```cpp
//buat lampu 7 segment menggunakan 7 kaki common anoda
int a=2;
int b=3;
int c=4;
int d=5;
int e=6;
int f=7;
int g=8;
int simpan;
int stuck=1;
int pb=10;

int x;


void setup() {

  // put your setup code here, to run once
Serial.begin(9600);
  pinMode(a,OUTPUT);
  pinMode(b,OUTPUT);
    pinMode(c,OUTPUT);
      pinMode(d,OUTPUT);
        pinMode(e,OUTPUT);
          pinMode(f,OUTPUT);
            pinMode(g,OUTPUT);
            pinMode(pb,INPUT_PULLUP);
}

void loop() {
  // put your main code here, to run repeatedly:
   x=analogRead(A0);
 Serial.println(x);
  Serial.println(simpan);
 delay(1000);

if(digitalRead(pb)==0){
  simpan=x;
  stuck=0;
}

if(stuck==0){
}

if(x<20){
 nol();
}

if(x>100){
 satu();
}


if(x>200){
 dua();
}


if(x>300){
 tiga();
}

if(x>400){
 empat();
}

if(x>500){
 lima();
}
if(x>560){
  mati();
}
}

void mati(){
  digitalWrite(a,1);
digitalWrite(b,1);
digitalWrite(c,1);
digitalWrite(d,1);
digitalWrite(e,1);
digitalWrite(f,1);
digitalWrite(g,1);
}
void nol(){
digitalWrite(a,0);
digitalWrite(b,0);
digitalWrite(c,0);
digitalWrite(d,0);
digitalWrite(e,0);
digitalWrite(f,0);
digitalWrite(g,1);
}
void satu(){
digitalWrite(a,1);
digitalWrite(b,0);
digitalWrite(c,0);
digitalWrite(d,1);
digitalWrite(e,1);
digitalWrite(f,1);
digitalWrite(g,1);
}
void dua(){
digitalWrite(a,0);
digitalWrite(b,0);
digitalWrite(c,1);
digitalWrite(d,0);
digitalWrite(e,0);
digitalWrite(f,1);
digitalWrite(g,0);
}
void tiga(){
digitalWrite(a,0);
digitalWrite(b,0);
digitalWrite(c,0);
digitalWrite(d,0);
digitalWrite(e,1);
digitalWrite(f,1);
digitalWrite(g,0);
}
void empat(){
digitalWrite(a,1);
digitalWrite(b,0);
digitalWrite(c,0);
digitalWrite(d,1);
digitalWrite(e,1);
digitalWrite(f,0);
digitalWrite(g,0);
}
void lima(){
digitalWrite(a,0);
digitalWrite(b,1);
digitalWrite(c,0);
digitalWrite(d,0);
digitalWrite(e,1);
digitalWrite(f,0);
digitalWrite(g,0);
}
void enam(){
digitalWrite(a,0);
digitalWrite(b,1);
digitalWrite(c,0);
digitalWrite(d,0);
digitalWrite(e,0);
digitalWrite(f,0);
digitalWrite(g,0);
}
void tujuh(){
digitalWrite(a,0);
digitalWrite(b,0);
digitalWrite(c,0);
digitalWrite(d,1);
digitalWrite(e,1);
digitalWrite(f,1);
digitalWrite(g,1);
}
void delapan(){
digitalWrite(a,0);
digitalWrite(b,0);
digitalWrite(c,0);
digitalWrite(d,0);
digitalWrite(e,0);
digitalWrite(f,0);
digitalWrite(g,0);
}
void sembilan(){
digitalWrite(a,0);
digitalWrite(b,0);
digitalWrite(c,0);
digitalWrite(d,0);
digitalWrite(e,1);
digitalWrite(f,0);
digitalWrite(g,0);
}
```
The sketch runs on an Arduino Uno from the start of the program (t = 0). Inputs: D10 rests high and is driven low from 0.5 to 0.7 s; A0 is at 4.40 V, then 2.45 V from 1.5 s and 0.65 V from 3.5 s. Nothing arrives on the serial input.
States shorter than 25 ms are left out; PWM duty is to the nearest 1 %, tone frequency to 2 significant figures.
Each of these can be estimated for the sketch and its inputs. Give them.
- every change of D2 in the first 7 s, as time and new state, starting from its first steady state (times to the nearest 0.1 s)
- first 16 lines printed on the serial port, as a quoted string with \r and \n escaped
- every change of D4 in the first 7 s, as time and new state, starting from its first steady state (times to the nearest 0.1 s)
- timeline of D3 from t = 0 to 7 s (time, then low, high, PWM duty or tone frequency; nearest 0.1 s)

0 s low; 1 s high; 3 s low; 5 s high
"901\r\n0\r\n901\r\n0\r\n501\r\n0\r\n501\r\n0\r\n133\r\n0\r\n133\r\n0\r\n133\r\n0\r\n133\r\n0\r\n"
0 s low; 1 s high; 3 s low
0 s low; 1 s high; 5 s low
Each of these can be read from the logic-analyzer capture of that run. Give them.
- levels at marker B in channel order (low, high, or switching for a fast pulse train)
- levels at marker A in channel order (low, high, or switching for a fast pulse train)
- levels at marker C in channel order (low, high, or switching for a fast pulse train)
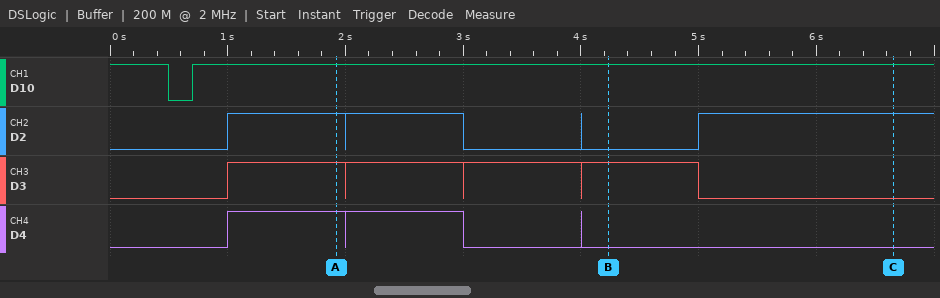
D10 high, D2 low, D3 high, D4 low
D10 high, D2 high, D3 high, D4 high
D10 high, D2 high, D3 low, D4 low
